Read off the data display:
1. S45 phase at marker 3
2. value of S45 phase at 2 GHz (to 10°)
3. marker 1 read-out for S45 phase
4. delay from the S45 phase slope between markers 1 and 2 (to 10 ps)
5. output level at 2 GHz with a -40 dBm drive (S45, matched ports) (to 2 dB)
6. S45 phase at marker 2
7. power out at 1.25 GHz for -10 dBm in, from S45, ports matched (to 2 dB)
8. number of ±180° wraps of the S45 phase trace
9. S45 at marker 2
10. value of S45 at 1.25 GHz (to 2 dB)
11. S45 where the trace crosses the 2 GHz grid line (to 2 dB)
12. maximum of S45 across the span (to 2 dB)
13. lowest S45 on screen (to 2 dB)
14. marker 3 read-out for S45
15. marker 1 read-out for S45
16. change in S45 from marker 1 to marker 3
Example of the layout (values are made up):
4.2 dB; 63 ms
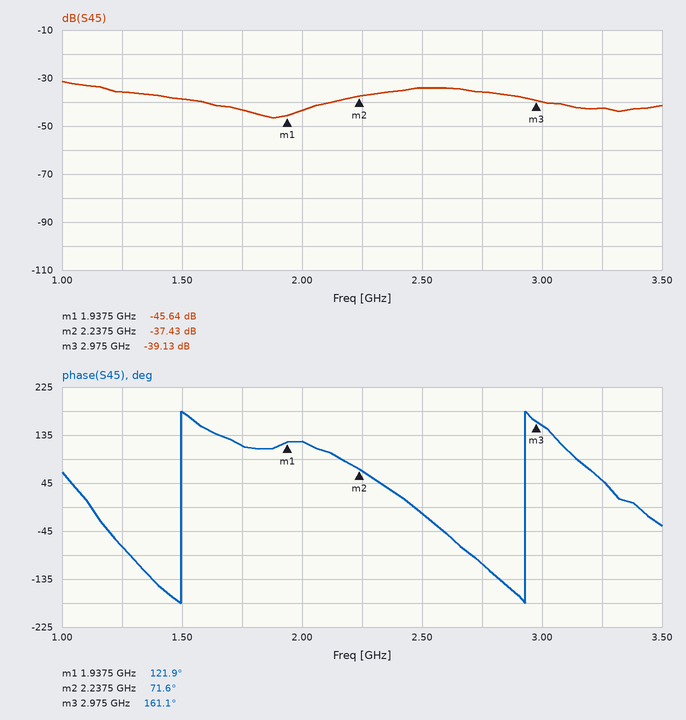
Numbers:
161.1°; 120°; 121.9°; 470 ps; -84 dBm; 71.6°; -46 dBm; 2; -37.43 dB; -36 dB; -44 dB; -32 dB; -46 dB; -39.13 dB; -45.64 dB; 6.51 dB
